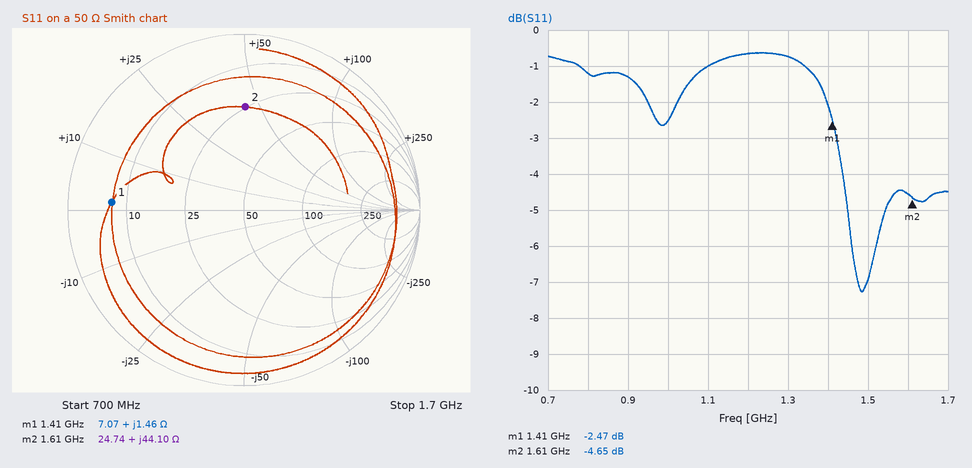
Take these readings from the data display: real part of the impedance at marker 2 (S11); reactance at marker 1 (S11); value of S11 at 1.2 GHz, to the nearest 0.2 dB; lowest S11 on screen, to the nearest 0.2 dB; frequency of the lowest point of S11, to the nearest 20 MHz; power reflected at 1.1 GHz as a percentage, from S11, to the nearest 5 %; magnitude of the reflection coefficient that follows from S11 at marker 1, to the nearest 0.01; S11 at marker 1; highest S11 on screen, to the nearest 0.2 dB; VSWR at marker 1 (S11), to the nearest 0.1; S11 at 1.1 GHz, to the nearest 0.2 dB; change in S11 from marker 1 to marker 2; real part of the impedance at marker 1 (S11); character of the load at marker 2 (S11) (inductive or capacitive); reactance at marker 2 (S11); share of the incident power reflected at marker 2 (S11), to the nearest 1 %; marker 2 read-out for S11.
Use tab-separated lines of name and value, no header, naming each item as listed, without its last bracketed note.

real part of the impedance at marker 2	24.74 Ω
reactance at marker 1	+1.46 Ω
value of S11 at 1.2 GHz, to the nearest 0.2 dB	-0.6 dB
lowest S11 on screen, to the nearest 0.2 dB	-7.2 dB
frequency of the lowest point of S11, to the nearest 20 MHz	1.48 GHz
power reflected at 1.1 GHz as a percentage, from S11, to the nearest 5 %	80 %
magnitude of the reflection coefficient that follows from S11 at marker 1, to the nearest 0.01	0.75
S11 at marker 1	-2.47 dB
highest S11 on screen, to the nearest 0.2 dB	-0.6 dB
VSWR at marker 1 (S11), to the nearest 0.1	7.1
S11 at 1.1 GHz, to the nearest 0.2 dB	-1.0 dB
change in S11 from marker 1 to marker 2	-2.18 dB
real part of the impedance at marker 1	7.07 Ω
character of the load at marker 2 (S11)	inductive
reactance at marker 2	+44.10 Ω
share of the incident power reflected at marker 2 (S11), to the nearest 1 %	34 %
marker 2 read-out for S11	-4.65 dB
